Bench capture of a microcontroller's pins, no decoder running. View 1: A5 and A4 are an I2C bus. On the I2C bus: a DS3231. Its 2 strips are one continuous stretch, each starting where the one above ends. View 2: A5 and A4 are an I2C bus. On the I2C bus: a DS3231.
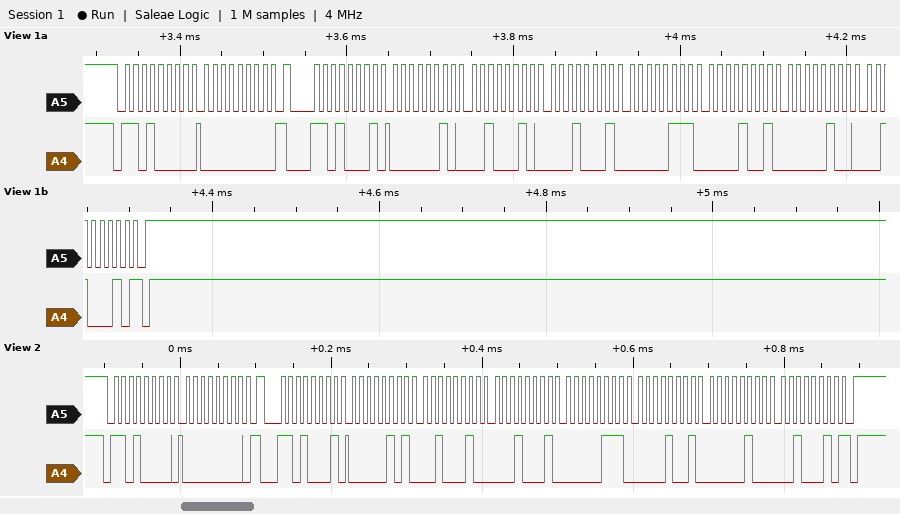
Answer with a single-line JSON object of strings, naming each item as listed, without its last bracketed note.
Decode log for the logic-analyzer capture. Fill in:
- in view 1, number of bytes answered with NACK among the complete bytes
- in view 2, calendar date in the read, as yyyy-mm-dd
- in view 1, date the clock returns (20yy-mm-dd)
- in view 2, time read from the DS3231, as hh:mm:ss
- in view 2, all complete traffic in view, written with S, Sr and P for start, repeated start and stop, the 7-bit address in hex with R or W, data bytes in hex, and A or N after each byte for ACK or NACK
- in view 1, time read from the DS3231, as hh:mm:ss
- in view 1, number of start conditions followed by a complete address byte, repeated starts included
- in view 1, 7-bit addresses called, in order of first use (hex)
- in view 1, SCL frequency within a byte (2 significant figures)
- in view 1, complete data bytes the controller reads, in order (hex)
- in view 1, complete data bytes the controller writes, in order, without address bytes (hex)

{"in view 1, number of bytes answered with NACK among the complete bytes": "1", "in view 2, calendar date in the read, as yyyy-mm-dd": "2022-04-09", "in view 1, date the clock returns": "2022-04-09", "in view 2, time read from the DS3231, as hh:mm:ss": "11:22:05", "in view 2, all complete traffic in view, written with S, Sr and P for start, repeated start and stop, the 7-bit address in hex with R or W, data bytes in hex, and A or N after each byte for ACK or NACK": "S 68W A 00 A Sr 68R A 05 A 22 A 11 A 07 A 09 A 04 A 22 N P", "in view 1, time read from the DS3231, as hh:mm:ss": "11:22:02", "in view 1, number of start conditions followed by a complete address byte, repeated starts included": "2", "in view 1, 7-bit addresses called, in order of first use": "0x68", "in view 1, SCL frequency within a byte": "100 kHz", "in view 1, complete data bytes the controller reads, in order": "02 22 11 07 09 04 22", "in view 1, complete data bytes the controller writes, in order, without address bytes": "00"}
